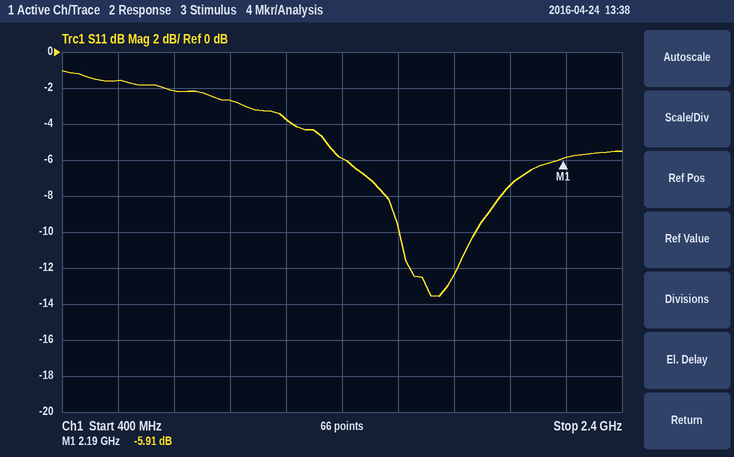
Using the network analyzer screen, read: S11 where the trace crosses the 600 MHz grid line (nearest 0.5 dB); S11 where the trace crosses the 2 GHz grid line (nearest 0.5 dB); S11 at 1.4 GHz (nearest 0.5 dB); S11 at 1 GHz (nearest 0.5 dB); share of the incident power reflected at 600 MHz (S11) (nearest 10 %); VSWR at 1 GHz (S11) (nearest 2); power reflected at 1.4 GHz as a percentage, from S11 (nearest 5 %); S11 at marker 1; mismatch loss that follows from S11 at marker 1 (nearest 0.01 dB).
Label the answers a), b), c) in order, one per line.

a) -1.5 dB
b) -7.5 dB
c) -6.0 dB
d) -2.5 dB
e) 70 %
f) 6
g) 25 %
h) -5.91 dB
i) 1.29 dB
